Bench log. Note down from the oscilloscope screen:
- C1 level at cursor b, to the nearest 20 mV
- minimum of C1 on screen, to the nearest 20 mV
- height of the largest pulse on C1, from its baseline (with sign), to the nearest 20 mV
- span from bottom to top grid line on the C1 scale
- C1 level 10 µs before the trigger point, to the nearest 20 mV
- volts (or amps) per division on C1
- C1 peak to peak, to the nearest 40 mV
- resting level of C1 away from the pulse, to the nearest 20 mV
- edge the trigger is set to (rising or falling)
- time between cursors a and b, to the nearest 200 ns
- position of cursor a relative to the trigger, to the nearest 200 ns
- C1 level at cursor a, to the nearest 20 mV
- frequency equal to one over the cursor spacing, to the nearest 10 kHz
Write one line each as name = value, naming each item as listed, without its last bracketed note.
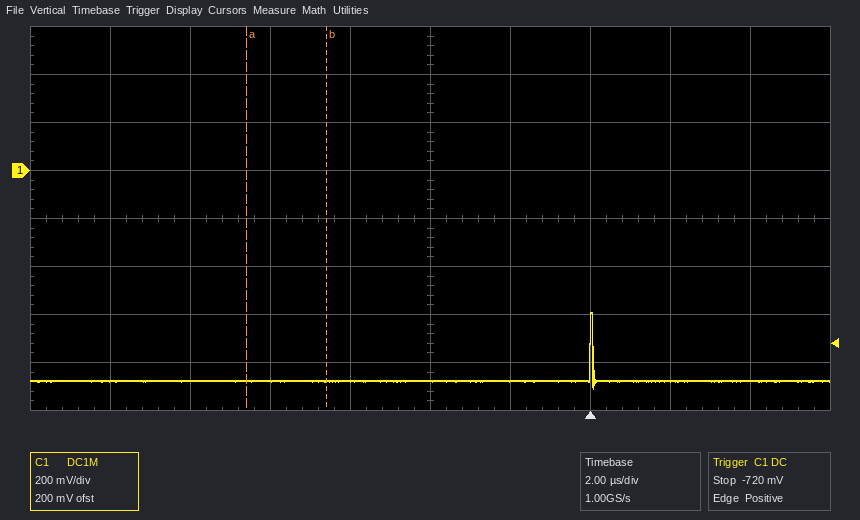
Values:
C1 level at cursor b, to the nearest 20 mV = -880 mV
minimum of C1 on screen, to the nearest 20 mV = -900 mV
height of the largest pulse on C1, from its baseline (with sign), to the nearest 20 mV = +280 mV
span from bottom to top grid line on the C1 scale = 1.6 V
C1 level 10 µs before the trigger point, to the nearest 20 mV = -880 mV
volts (or amps) per division on C1 = 200 mV
C1 peak to peak, to the nearest 40 mV = 320 mV
resting level of C1 away from the pulse, to the nearest 20 mV = -880 mV
edge the trigger is set to = rising
time between cursors a and b, to the nearest 200 ns = 2.0 µs
position of cursor a relative to the trigger, to the nearest 200 ns = -8.6 µs
C1 level at cursor a, to the nearest 20 mV = -880 mV
frequency equal to one over the cursor spacing, to the nearest 10 kHz = 500 kHz
